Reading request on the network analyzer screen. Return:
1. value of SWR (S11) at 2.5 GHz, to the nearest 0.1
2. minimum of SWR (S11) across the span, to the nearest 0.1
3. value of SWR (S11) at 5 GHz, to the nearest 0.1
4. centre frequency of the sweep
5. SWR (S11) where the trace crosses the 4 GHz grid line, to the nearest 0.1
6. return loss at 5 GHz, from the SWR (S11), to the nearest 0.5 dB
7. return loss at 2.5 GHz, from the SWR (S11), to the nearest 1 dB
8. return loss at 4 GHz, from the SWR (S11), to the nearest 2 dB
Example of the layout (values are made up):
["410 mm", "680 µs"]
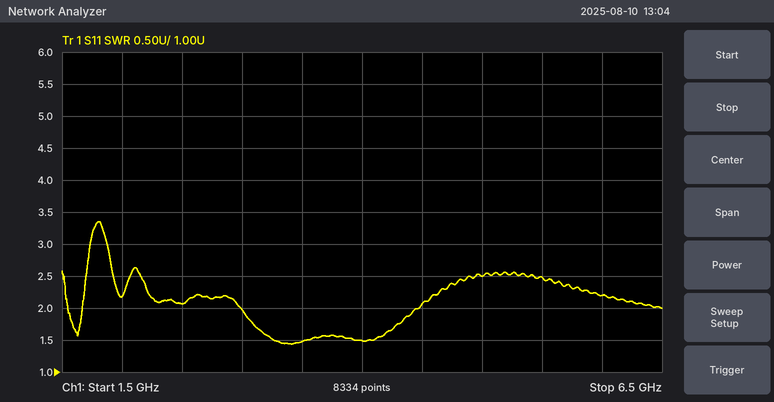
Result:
["2.1", "1.4", "2.5", "4 GHz", "1.5", "7.5 dB", "9 dB", "14 dB"]
